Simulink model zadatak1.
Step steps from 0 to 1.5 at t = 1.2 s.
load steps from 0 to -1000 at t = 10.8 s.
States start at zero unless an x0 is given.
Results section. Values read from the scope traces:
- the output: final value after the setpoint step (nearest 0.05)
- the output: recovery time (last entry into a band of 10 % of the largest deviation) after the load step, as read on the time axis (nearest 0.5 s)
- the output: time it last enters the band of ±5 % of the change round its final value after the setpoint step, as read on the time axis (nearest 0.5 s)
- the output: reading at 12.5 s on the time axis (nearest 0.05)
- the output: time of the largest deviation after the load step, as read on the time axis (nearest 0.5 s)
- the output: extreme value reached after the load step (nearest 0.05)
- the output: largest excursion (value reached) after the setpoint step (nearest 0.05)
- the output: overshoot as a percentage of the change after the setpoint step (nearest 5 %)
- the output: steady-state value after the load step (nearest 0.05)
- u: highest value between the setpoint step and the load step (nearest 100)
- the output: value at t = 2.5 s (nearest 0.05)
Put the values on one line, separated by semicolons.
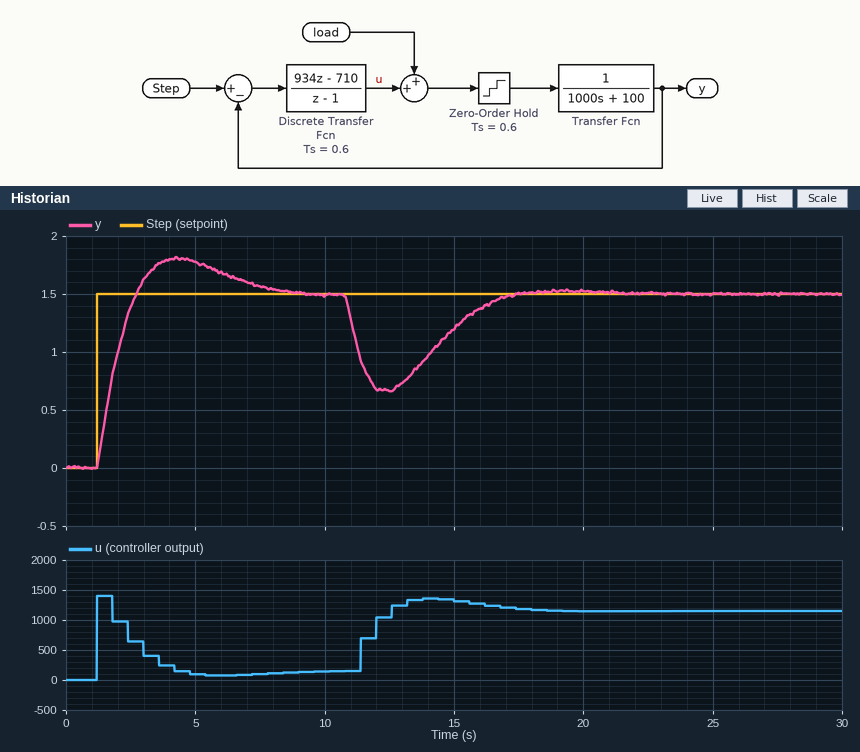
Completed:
1.50; 16.5 s; 7.5 s; 0.65; 12.5 s; 0.65; 1.80; 20 %; 1.50; 1400; 1.40
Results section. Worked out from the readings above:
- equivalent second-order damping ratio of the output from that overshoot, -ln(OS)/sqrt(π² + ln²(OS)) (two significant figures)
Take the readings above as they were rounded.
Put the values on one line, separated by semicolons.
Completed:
0.46
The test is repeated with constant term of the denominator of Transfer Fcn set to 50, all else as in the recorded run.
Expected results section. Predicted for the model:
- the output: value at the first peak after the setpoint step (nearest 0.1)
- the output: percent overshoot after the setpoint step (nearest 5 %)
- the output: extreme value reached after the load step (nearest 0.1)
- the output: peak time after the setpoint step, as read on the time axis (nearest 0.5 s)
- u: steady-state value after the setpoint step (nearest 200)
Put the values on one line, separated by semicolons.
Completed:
1.9; 25 %; 0.6; 4.0 s; 0
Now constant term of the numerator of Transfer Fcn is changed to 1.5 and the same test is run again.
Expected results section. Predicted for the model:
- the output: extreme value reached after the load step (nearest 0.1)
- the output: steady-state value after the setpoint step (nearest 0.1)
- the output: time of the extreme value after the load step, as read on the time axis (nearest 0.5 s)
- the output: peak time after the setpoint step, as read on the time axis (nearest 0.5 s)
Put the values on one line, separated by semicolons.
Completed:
0.5; 1.5; 12.0 s; 3.0 s
